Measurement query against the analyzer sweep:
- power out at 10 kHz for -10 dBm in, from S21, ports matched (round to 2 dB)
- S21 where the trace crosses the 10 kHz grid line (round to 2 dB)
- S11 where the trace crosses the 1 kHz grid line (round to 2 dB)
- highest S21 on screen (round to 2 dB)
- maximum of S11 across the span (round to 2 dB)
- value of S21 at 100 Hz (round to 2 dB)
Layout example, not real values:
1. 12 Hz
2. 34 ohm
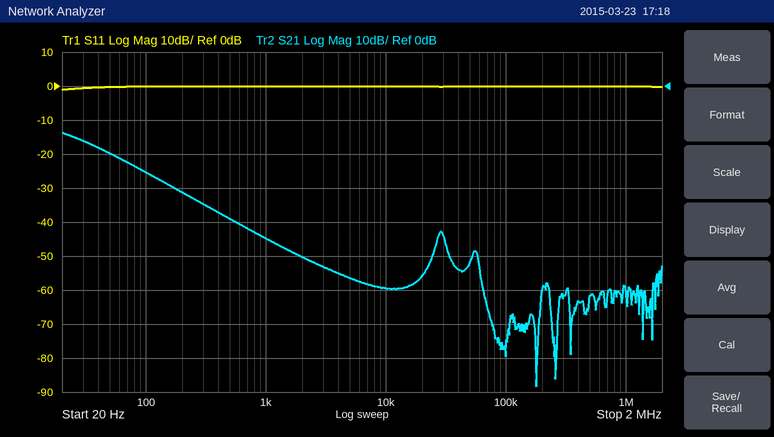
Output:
1. -70 dBm
2. -60 dB
3. 0 dB
4. -14 dB
5. 0 dB
6. -26 dB
